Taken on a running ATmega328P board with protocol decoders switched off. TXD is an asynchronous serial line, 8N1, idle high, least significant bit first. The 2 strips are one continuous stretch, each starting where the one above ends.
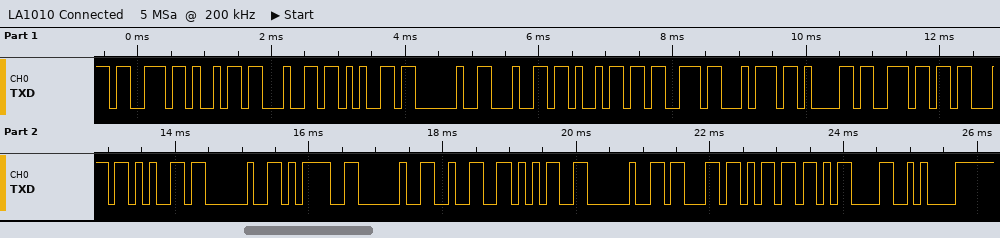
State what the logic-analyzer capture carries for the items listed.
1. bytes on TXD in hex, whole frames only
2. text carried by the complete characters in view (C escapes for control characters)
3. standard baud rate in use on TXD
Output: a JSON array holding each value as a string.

["0x73 0x69 0x64 0x65 0x20 0x64 0x69 0x73 0x74 0x61 0x6E 0x63 0x65 0x20 0x3D 0x20 0x32 0x35 0x20 0x63 0x6D 0x0D 0x0A", "\"side distance = 25 cm\\r\\n\"", "9600 baud"]
